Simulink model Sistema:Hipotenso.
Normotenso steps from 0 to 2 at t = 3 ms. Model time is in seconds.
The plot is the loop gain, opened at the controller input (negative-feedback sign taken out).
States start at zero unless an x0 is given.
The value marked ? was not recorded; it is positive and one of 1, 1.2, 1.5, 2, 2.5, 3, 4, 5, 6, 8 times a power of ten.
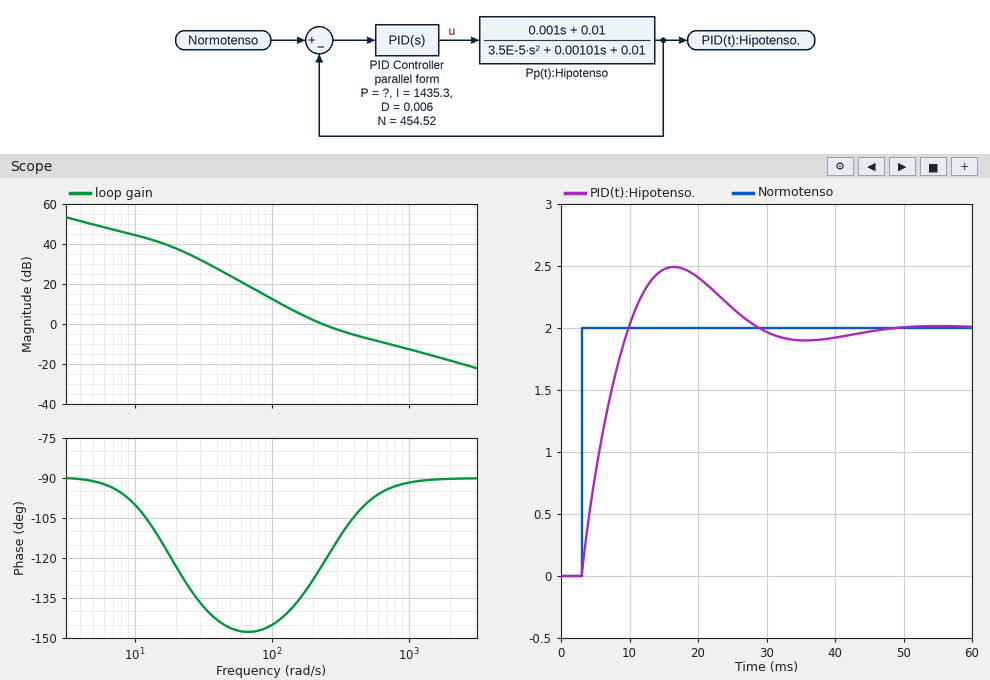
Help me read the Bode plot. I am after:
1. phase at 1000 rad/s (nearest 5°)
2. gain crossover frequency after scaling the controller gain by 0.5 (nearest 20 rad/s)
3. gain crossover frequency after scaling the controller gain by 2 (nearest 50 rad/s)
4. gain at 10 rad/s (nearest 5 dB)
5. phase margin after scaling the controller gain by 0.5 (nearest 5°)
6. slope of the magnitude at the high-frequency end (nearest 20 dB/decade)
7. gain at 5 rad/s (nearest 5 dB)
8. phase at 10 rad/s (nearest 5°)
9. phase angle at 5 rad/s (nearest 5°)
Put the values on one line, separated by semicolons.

-90°; 160 rad/s; 450 rad/s; 45 dB; 45°; -20 dB/decade; 50 dB; -100°; -90°
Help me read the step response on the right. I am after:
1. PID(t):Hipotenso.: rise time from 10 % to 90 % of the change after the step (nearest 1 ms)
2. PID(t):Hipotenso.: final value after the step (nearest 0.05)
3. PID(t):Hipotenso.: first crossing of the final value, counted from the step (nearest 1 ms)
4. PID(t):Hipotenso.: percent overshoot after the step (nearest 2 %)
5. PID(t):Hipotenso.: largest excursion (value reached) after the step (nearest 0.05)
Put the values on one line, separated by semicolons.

5 ms; 2.00; 7 ms; 24 %; 2.50
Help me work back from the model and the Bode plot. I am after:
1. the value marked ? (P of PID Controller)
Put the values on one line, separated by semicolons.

6
